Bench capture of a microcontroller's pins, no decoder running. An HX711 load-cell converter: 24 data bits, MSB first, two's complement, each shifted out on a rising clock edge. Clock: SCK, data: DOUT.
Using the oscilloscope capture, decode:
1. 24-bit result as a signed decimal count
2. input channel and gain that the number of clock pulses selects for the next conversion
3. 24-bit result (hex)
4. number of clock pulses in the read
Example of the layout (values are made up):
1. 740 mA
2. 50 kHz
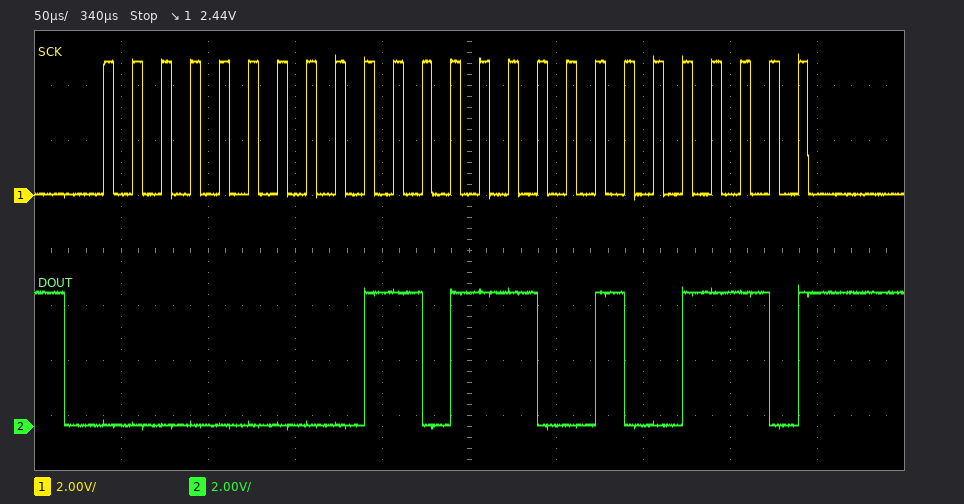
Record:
1. 28238
2. channel A, gain 128
3. 0x006E4E
4. 25
